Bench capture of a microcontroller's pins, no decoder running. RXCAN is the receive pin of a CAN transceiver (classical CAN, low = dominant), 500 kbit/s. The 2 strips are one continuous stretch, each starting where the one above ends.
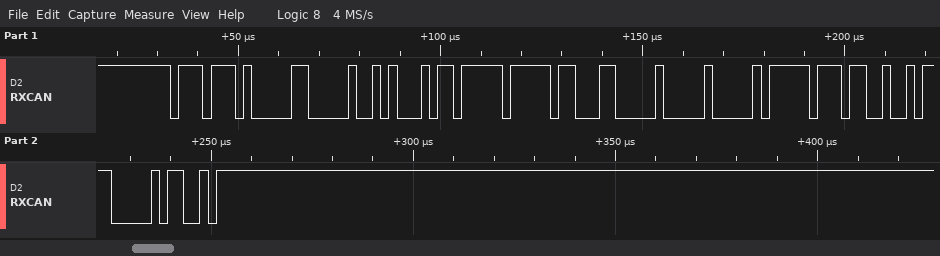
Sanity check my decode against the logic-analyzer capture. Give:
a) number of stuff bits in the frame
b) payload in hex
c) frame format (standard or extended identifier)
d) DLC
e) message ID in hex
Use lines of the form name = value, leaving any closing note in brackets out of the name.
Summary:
number of stuff bits in the frame = 9
payload in hex = 0A 2D FF E3 00 00 FF 64
frame format = standard
DLC = 8
message ID in hex = 0x774
